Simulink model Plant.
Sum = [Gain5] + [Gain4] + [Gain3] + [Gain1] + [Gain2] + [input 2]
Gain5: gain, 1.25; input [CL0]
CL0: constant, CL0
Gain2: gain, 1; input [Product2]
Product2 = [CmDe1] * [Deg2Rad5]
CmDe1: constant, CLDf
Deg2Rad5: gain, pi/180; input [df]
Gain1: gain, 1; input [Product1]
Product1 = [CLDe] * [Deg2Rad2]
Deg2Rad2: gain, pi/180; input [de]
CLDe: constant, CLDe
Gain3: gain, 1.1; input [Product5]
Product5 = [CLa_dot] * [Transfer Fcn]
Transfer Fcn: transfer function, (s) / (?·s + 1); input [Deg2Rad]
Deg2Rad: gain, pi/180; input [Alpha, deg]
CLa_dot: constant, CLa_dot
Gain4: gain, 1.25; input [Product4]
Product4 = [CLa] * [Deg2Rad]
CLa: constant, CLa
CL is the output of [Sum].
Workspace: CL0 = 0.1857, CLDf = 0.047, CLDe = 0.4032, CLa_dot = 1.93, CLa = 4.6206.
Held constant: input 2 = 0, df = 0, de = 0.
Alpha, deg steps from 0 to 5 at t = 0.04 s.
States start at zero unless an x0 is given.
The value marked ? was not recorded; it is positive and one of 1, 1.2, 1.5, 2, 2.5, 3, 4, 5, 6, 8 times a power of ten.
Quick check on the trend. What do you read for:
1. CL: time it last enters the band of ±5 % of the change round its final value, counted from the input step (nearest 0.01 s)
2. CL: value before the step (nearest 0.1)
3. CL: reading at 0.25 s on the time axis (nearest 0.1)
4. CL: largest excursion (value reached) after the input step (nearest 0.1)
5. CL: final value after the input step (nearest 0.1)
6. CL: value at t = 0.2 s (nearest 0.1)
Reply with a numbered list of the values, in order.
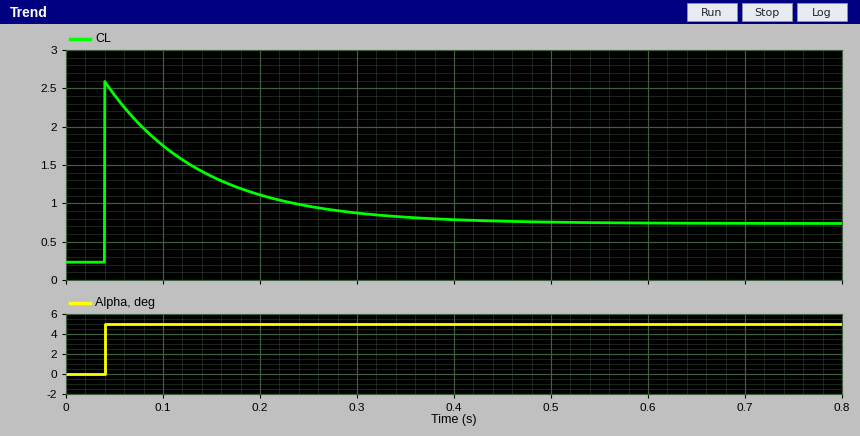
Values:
1. 0.43 s
2. 0.2
3. 1.0
4. 2.6
5. 0.7
6. 1.1
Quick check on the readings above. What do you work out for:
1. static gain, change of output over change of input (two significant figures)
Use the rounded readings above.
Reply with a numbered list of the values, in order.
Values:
1. 0.10
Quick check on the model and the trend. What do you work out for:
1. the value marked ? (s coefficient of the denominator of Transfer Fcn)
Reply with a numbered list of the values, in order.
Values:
1. 0.1
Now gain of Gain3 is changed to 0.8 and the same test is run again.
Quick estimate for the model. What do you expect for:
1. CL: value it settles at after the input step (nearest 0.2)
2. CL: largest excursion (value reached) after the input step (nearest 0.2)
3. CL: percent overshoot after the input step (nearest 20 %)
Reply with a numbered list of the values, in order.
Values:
1. 0.8
2. 2.0
3. 260 %
